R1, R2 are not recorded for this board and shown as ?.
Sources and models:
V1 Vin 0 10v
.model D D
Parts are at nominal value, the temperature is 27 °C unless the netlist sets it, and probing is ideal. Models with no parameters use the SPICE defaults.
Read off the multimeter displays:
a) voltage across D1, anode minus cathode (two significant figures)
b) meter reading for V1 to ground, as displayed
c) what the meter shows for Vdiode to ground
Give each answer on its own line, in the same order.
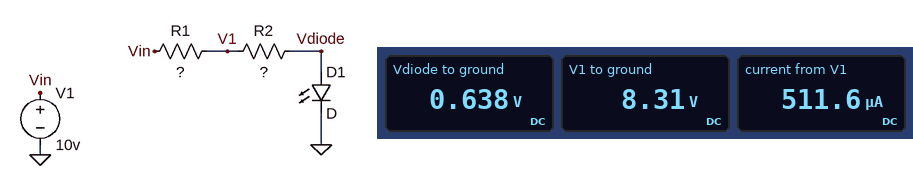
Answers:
640 mV
8.31 V
0.638 V
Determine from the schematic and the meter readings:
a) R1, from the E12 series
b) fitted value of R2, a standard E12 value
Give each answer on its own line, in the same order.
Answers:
3.3 kΩ
15 kΩ
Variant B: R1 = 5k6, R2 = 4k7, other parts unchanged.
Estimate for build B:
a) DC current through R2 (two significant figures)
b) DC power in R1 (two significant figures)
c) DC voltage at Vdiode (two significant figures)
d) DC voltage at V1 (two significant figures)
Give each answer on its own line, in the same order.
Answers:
910 µA
4.6 mW
650 mV
4.9 V
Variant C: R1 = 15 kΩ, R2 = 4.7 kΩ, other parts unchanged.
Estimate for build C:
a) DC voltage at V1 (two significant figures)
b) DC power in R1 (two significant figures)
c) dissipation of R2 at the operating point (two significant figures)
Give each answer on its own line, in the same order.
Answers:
2.9 V
3.4 mW
1.1 mW
